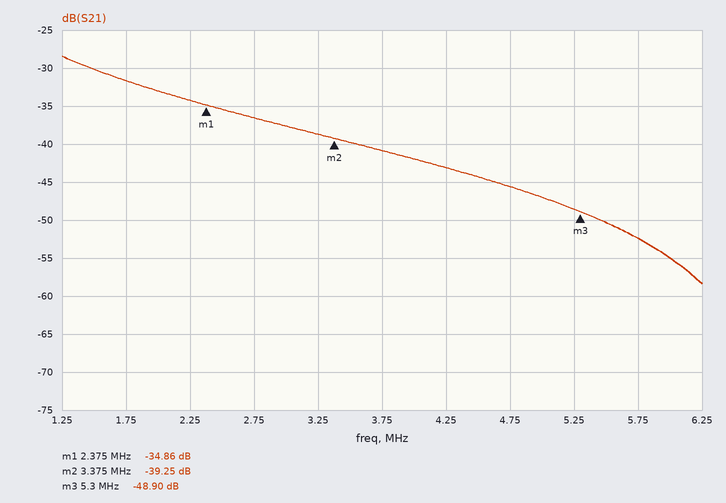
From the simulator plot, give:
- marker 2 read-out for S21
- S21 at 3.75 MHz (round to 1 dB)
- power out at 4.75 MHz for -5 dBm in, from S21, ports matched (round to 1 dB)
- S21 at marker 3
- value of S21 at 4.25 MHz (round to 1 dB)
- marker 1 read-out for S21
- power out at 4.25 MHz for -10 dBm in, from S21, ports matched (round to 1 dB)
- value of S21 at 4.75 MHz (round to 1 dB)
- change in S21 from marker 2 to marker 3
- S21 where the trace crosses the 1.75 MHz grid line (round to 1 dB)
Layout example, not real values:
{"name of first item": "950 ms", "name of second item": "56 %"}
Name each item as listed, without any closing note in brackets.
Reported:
{"marker 2 read-out for S21": "-39.25 dB", "S21 at 3.75 MHz": "-41 dB", "power out at 4.75 MHz for -5 dBm in, from S21, ports matched": "-51 dBm", "S21 at marker 3": "-48.90 dB", "value of S21 at 4.25 MHz": "-43 dB", "marker 1 read-out for S21": "-34.86 dB", "power out at 4.25 MHz for -10 dBm in, from S21, ports matched": "-53 dBm", "value of S21 at 4.75 MHz": "-46 dB", "change in S21 from marker 2 to marker 3": "-9.65 dB", "S21 where the trace crosses the 1.75 MHz grid line": "-32 dB"}
